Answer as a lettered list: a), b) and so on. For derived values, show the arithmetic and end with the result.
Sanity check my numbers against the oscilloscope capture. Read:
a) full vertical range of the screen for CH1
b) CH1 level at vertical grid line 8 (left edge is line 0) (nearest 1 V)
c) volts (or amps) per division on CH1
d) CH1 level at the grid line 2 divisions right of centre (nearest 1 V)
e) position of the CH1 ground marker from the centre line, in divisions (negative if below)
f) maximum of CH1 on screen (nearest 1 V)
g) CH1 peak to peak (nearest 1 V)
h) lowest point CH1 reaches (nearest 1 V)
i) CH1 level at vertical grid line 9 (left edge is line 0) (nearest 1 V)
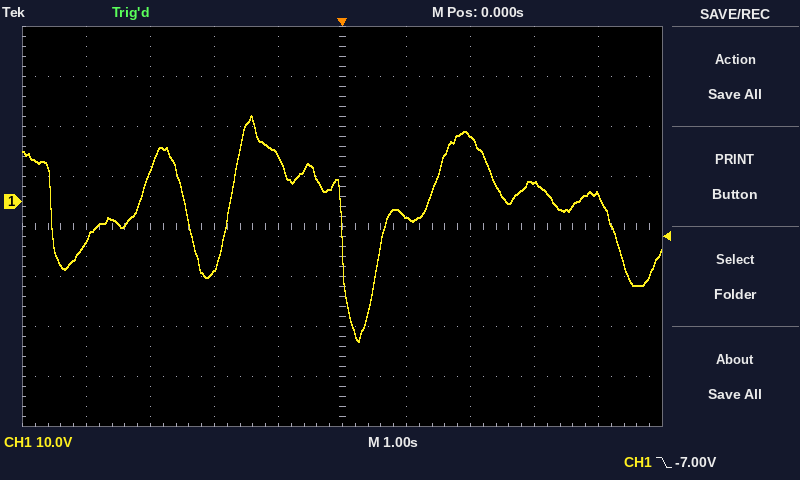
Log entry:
a) 80 V
b) 4 V
c) 10 V
d) 13 V
e) +0.5 div
f) 17 V
g) 17 V − (-28 V) = 45 V
h) -28 V
i) 1 V
